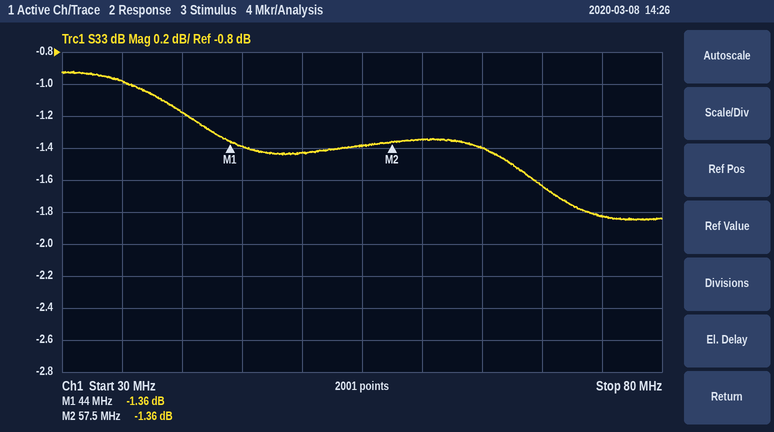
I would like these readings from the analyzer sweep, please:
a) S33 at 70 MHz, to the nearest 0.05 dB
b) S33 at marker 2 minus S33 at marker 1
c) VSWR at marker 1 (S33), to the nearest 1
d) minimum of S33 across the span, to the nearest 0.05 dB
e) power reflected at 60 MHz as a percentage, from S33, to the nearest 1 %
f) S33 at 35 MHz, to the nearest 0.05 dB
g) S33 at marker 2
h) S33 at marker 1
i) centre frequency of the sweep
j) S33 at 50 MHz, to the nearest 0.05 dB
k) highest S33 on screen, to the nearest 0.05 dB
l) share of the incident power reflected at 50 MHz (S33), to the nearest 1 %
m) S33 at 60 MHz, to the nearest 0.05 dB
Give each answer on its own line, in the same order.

-1.65 dB
0.00 dB
13
-1.85 dB
73 %
-1.00 dB
-1.36 dB
-1.36 dB
55 MHz
-1.45 dB
-0.90 dB
72 %
-1.35 dB
